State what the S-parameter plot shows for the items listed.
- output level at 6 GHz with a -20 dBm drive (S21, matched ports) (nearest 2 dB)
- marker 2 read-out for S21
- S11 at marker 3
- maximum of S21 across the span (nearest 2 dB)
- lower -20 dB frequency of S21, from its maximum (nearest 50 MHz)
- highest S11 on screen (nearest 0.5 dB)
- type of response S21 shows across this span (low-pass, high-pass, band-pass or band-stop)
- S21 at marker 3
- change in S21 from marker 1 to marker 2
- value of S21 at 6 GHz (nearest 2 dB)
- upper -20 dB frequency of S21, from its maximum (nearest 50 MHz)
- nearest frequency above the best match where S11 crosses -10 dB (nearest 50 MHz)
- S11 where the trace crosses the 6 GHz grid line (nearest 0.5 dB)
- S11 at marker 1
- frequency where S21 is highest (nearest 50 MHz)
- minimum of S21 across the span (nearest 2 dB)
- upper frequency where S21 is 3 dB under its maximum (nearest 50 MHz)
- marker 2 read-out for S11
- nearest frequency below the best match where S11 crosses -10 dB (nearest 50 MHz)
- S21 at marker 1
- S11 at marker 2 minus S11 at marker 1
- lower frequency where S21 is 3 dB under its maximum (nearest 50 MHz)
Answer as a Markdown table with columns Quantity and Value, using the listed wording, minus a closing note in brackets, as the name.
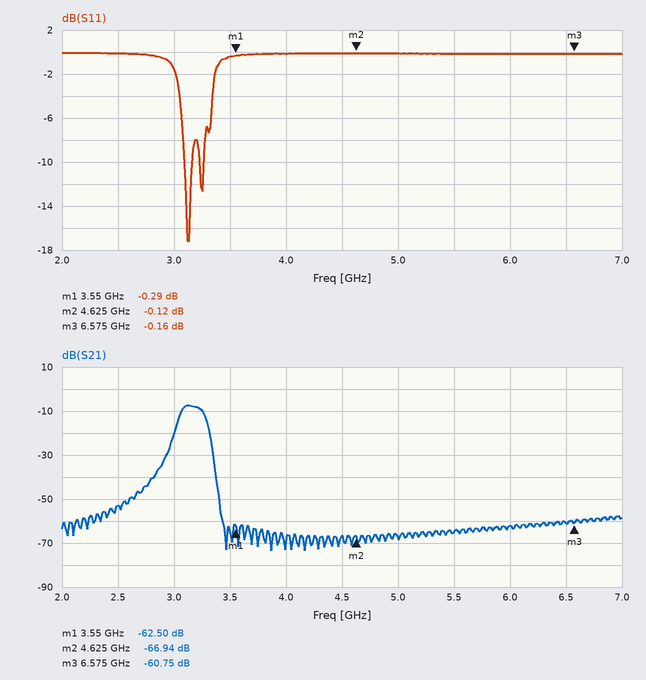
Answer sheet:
| Quantity | Value |
|---|---|
| output level at 6 GHz with a -20 dBm drive (S21, matched ports) | -82 dBm |
| marker 2 read-out for S21 | -66.94 dB |
| S11 at marker 3 | -0.16 dB |
| maximum of S21 across the span | -8 dB |
| lower -20 dB frequency of S21, from its maximum | 2.95 GHz |
| highest S11 on screen | 0.0 dB |
| type of response S21 shows across this span | band-pass |
| S21 at marker 3 | -60.75 dB |
| change in S21 from marker 1 to marker 2 | -4.44 dB |
| value of S21 at 6 GHz | -62 dB |
| upper -20 dB frequency of S21, from its maximum | 3.35 GHz |
| nearest frequency above the best match where S11 crosses -10 dB | 3.15 GHz |
| S11 where the trace crosses the 6 GHz grid line | 0.0 dB |
| S11 at marker 1 | -0.29 dB |
| frequency where S21 is highest | 3.10 GHz |
| minimum of S21 across the span | -74 dB |
| upper frequency where S21 is 3 dB under its maximum | 3.25 GHz |
| marker 2 read-out for S11 | -0.12 dB |
| nearest frequency below the best match where S11 crosses -10 dB | 3.10 GHz |
| S21 at marker 1 | -62.50 dB |
| S11 at marker 2 minus S11 at marker 1 | 0.17 dB |
| lower frequency where S21 is 3 dB under its maximum | 3.05 GHz |
